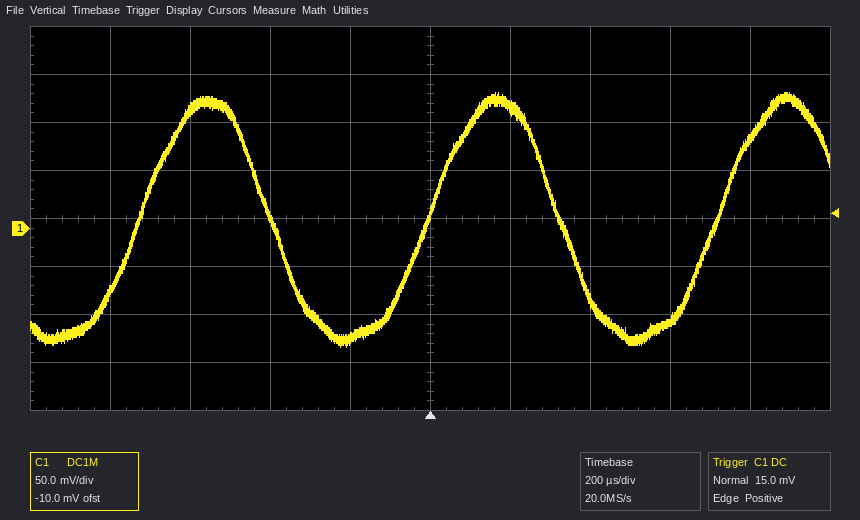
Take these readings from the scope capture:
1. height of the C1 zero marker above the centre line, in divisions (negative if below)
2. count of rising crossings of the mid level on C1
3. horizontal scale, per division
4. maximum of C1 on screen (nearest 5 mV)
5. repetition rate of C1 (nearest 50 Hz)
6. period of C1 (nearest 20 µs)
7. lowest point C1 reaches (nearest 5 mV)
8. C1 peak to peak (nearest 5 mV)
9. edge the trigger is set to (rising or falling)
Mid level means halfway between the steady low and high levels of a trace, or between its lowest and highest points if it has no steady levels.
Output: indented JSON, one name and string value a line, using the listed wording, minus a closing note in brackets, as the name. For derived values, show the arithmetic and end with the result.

{
  "height of the C1 zero marker above the centre line, in divisions": "-0.2 div",
  "count of rising crossings of the mid level on C1": "3",
  "horizontal scale, per division": "200 µs",
  "maximum of C1 on screen": "140 mV",
  "repetition rate of C1": "1 / 720 µs ≈ 1.39 kHz, so 1.40 kHz to the nearest 50 Hz",
  "period of C1": "720 µs",
  "lowest point C1 reaches": "-125 mV",
  "C1 peak to peak": "140 mV − (-125 mV) = 265 mV",
  "edge the trigger is set to": "rising"
}
